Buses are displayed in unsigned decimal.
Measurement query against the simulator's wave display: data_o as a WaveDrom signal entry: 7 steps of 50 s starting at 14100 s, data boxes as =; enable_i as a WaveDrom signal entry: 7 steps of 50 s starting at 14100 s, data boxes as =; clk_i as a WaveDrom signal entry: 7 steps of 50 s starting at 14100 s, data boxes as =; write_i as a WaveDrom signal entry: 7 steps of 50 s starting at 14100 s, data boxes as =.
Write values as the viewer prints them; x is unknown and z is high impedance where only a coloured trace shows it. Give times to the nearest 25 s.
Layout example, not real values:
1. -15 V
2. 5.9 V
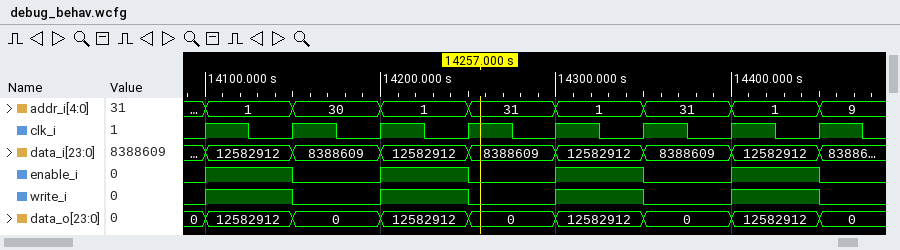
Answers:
1. {name: 'data_o', wave: '=======', data: '12582912 0 12582912 0 12582912 0 12582912'}
2. {name: 'enable_i', wave: '1010101'}
3. {name: 'clk_i', wave: 'p......'}
4. {name: 'write_i', wave: '1010101'}
